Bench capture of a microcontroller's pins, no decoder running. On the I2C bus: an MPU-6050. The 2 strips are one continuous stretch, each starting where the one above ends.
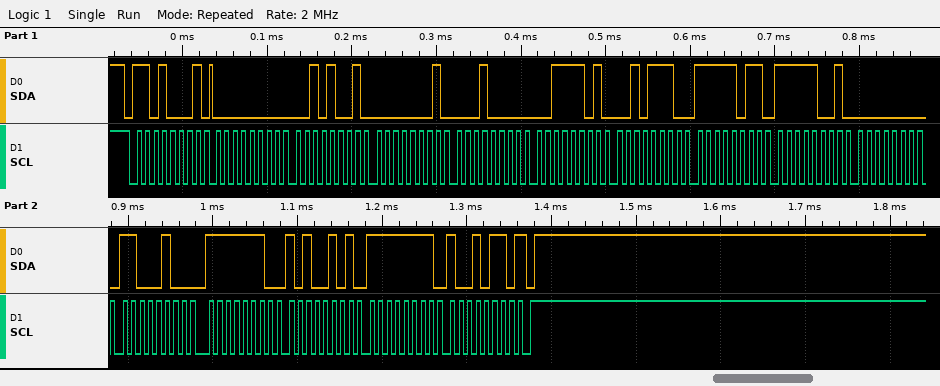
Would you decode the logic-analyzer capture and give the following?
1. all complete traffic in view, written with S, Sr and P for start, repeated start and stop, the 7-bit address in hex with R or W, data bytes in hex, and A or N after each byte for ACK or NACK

S 68R A 00 A 29 A 01 A 10 A 3D A 2E A FB A F9 A 00 A C4 A FE A A5 A FF A 96 N P
